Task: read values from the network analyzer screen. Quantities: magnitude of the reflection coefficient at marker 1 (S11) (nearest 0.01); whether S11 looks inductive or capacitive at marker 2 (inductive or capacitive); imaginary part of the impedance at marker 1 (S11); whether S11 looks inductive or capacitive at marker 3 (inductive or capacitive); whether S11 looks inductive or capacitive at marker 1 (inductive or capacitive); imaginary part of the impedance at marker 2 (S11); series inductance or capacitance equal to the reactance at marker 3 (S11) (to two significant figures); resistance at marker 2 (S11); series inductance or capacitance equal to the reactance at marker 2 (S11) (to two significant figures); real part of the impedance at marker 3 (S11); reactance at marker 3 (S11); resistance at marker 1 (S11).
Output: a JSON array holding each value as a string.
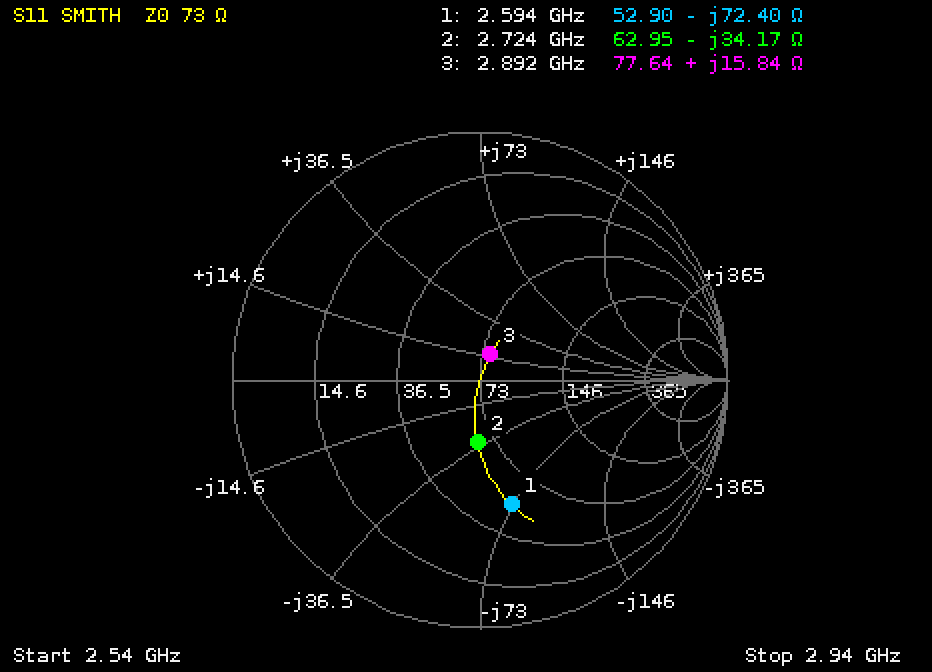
["0.52", "capacitive", "-72.40 Ω", "inductive", "capacitive", "-34.17 Ω", "870 pH", "62.95 Ω", "1.7 pF", "77.64 Ω", "+15.84 Ω", "52.90 Ω"]
